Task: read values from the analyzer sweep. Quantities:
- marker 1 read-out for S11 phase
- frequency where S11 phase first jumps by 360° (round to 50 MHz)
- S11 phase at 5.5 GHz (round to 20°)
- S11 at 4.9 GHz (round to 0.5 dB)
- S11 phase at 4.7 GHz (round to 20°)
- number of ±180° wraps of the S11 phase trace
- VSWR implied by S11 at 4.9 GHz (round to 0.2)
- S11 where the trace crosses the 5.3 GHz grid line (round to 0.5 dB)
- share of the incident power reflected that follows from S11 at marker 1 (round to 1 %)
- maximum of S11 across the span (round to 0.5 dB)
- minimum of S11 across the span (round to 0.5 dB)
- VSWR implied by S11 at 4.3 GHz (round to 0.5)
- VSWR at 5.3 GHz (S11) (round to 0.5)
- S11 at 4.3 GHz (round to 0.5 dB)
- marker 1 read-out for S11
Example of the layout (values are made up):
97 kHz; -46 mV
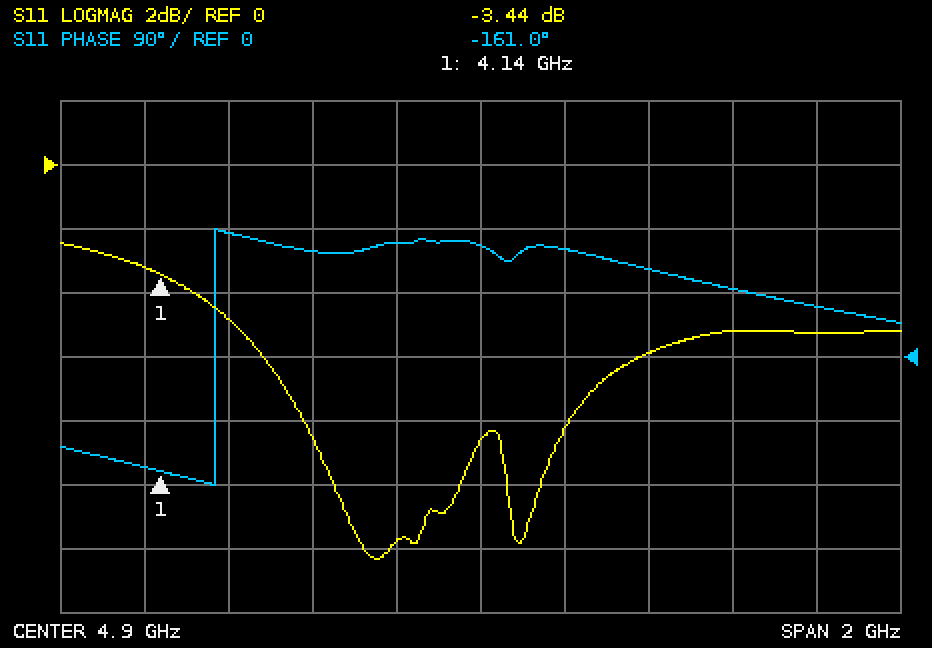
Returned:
-161.0°; 4.25 GHz; 100°; -8.5 dB; 160°; 1; 2.2; -6.0 dB; 45 %; -2.5 dB; -12.5 dB; 3.5; 3.0; -5.0 dB; -3.44 dB
